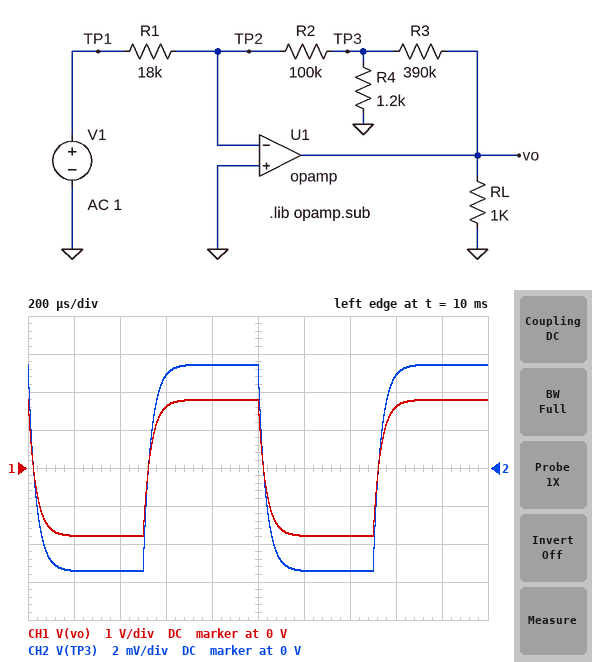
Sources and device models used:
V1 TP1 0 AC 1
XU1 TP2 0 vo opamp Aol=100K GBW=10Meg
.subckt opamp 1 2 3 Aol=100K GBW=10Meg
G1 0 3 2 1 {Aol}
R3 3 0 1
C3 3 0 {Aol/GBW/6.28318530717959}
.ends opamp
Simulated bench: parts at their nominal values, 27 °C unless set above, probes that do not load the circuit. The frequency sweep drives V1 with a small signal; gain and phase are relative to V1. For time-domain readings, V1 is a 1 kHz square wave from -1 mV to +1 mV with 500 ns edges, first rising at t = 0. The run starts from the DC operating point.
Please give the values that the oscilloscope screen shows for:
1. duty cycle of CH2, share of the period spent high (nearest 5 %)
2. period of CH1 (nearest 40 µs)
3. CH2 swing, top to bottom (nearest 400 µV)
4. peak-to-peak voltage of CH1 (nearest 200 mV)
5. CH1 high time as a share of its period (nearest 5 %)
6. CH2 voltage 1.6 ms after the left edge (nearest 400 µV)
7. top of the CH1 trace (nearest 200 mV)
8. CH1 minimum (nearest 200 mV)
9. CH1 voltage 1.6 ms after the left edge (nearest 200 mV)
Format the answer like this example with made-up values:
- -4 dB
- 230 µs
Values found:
- 50 %
- 1.00 ms
- 10.8 mV
- 3.6 V
- 50 %
- 4.8 mV
- 1.8 V
- -1.8 V
- 1.6 V
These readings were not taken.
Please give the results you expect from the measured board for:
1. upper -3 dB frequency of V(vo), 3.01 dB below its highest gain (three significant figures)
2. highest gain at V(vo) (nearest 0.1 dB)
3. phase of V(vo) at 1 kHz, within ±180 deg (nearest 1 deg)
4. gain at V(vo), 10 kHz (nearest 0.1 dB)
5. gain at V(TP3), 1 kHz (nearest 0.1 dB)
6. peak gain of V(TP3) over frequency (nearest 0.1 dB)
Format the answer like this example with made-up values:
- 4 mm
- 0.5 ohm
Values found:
- 4.73 kHz
- 65.1 dB
- 168 deg
- 57.7 dB
- 14.5 dB
- 14.7 dB
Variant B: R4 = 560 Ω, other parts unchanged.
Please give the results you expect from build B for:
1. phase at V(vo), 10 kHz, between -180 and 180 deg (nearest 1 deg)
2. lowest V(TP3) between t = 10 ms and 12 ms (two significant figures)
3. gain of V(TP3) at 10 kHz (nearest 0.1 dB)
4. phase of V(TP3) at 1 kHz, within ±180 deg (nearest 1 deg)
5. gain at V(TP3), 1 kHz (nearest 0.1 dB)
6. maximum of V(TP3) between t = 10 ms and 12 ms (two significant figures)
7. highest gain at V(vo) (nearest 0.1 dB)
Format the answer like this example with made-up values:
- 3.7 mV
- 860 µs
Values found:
- 103 deg
- -5.3 mV
- 1.4 dB
- 156 deg
- 13.7 dB
- 5.3 mV
- 71.4 dB
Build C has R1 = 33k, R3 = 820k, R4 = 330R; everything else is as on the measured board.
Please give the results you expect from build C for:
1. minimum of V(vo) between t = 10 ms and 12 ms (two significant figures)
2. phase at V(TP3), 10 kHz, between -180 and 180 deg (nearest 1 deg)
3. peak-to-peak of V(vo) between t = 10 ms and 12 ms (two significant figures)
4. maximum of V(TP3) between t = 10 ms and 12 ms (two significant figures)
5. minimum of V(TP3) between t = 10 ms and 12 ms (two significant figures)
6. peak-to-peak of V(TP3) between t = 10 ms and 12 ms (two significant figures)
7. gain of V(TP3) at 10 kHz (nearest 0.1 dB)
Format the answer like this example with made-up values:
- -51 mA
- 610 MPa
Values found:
- -6.4 V
- 96 deg
- 13 V
- 2.6 mV
- -2.6 mV
- 5.2 mV
- -10.5 dB
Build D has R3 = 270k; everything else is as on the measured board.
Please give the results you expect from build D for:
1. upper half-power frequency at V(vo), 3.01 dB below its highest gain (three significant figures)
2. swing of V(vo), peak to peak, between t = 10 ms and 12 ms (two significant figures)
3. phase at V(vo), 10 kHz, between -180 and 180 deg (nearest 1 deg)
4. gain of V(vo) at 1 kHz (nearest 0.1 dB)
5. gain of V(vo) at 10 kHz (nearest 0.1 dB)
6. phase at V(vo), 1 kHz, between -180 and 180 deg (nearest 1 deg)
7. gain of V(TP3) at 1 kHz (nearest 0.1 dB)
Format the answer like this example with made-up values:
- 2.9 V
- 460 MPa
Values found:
- 6.78 kHz
- 2.5 V
- 124 deg
- 61.9 dB
- 56.9 dB
- 172 deg
- 14.7 dB
